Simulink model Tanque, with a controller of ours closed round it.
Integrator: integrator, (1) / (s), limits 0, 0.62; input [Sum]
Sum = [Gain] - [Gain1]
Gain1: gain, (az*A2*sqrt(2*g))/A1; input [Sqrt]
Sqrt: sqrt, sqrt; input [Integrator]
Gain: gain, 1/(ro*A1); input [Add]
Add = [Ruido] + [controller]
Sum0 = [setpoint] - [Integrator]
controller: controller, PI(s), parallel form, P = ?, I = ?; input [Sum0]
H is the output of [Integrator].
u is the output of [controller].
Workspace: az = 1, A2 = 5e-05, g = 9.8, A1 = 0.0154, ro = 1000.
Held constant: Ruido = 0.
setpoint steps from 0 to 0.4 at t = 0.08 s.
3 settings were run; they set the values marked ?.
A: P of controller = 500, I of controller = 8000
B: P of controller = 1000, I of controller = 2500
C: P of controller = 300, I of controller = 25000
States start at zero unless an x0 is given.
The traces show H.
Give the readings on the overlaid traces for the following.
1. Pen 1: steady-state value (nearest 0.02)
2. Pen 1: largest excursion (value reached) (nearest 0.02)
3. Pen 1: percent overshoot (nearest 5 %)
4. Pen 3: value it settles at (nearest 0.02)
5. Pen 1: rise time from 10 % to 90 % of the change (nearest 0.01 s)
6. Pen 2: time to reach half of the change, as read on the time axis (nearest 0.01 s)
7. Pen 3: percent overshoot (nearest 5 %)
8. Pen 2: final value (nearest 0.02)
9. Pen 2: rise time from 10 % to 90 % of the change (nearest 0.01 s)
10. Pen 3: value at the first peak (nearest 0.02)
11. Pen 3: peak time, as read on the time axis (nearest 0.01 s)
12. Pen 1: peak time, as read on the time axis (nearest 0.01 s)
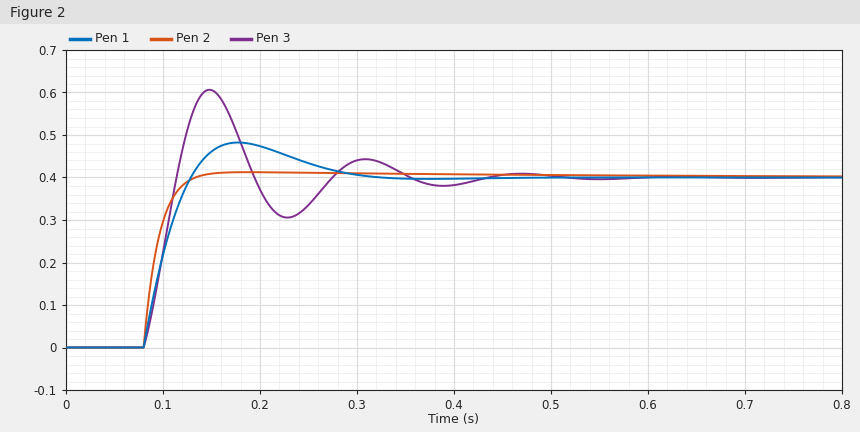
0.40
0.48
20 %
0.40
0.04 s
0.09 s
50 %
0.40
0.03 s
0.60
0.15 s
0.18 s
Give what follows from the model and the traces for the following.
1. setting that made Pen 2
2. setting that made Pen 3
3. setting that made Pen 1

B
C
A
